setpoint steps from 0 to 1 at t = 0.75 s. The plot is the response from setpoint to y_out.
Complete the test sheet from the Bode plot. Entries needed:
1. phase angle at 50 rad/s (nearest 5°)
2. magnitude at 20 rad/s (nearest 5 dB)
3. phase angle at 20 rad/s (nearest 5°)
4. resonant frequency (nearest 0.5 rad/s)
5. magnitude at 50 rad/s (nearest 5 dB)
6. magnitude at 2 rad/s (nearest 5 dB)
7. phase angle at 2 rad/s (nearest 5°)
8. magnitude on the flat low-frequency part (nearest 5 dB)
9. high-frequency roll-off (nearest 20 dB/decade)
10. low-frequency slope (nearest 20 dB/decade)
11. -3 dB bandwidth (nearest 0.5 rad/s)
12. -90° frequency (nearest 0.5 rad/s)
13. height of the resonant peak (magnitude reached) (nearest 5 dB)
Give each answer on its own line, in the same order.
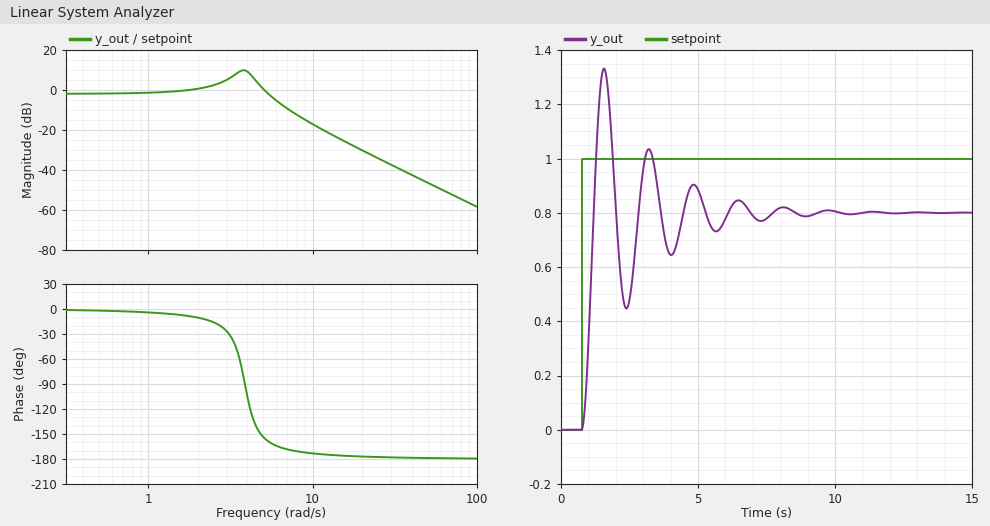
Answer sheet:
-180°
-30 dB
-175°
4.0 rad/s
-45 dB
0 dB
-10°
0 dB
-40 dB/decade
0 dB/decade
6.0 rad/s
4.0 rad/s
10 dB
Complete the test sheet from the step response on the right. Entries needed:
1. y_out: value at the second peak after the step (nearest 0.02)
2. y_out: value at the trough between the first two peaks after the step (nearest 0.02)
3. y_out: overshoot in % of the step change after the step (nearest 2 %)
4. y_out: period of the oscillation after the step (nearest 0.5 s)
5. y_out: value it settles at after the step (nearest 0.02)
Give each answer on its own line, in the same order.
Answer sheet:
1.04
0.44
66 %
1.5 s
0.80
